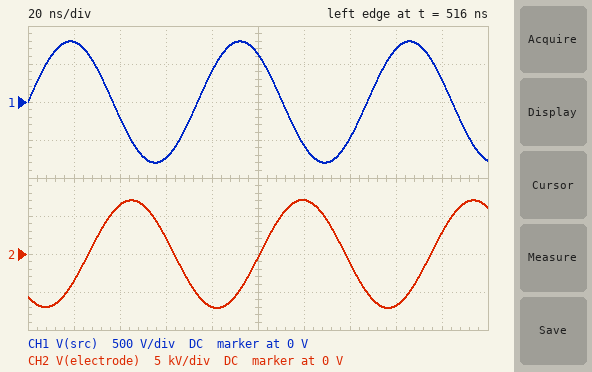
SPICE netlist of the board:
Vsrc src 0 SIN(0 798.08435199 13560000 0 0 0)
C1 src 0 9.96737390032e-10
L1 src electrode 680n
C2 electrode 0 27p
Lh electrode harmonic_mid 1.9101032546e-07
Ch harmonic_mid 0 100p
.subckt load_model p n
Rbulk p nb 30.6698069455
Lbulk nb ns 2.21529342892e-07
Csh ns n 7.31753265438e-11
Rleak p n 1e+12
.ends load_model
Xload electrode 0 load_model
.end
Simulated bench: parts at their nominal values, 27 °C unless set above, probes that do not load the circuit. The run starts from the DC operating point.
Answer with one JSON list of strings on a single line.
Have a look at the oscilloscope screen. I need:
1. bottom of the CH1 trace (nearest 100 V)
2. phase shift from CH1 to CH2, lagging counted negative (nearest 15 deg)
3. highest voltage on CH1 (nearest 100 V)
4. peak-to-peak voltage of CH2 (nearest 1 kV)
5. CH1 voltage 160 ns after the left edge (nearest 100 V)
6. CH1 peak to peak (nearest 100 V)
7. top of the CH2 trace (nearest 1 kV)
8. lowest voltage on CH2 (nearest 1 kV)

["-800 V", "-135 deg", "800 V", "14 kV", "700 V", "1.6 kV", "7 kV", "-7 kV"]
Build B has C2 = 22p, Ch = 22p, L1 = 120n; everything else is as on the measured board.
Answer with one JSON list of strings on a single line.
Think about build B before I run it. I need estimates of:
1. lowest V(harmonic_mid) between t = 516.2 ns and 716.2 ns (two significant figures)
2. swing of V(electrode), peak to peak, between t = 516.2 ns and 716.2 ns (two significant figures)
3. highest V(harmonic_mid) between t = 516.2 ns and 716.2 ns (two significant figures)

["-920 V", "1.8 kV", "920 V"]
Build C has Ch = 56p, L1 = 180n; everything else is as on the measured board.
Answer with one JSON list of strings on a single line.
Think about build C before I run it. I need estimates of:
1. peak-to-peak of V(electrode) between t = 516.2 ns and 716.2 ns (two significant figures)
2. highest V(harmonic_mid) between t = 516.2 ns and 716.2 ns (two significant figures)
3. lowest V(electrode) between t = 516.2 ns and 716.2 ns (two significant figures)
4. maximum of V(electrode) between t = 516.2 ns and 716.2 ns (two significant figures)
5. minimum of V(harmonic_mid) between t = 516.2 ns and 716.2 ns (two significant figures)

["2.0 kV", "1.1 kV", "-1.0 kV", "1.0 kV", "-1.1 kV"]
